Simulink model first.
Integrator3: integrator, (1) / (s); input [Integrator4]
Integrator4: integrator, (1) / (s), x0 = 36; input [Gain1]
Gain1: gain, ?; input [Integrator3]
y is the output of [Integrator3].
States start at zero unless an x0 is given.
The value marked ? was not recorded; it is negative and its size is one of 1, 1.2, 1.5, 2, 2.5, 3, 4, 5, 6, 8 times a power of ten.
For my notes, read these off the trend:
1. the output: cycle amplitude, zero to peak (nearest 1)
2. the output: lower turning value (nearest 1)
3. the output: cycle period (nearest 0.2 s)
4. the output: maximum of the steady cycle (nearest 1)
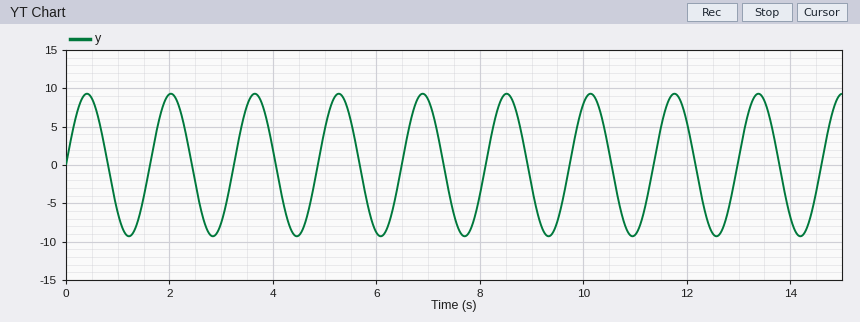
9
-9
1.6 s
9
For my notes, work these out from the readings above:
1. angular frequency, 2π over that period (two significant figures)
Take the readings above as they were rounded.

3.9 rad/s
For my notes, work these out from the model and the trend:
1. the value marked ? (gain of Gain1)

-15
